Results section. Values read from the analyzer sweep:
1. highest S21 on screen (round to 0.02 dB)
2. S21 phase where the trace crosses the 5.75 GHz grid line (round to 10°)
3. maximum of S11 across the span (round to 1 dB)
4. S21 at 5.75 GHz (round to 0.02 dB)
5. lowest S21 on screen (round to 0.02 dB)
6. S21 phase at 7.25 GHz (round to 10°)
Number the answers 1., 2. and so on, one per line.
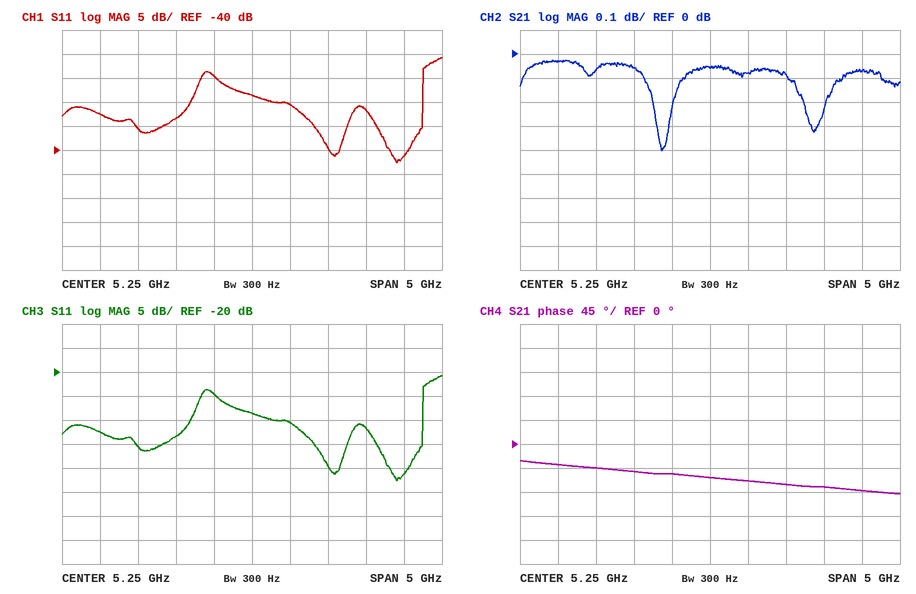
1. -0.02 dB
2. -70°
3. -21 dB
4. -0.08 dB
5. -0.40 dB
6. -90°
